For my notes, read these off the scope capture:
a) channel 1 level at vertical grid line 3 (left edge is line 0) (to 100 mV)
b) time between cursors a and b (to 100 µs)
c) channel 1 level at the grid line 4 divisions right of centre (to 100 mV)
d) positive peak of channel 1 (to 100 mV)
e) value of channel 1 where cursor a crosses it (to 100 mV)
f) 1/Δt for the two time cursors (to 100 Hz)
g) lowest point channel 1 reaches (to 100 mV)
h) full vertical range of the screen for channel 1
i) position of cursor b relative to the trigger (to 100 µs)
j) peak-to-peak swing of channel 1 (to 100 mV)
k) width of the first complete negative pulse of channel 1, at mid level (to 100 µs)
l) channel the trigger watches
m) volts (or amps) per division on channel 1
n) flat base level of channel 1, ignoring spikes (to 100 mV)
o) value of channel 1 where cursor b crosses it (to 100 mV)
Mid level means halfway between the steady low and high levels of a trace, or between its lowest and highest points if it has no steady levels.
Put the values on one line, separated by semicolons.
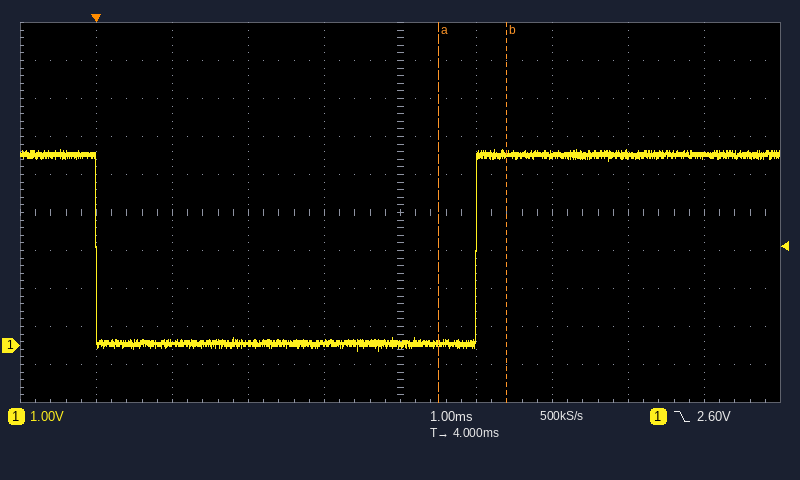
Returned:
100 mV; 900 µs; 5.0 V; 5.2 V; 100 mV; 1.1 kHz; -100 mV; 10 V; +5.4 ms; 5.3 V; 5.0 ms; channel 1; 1 V; 100 mV; 5.0 V
